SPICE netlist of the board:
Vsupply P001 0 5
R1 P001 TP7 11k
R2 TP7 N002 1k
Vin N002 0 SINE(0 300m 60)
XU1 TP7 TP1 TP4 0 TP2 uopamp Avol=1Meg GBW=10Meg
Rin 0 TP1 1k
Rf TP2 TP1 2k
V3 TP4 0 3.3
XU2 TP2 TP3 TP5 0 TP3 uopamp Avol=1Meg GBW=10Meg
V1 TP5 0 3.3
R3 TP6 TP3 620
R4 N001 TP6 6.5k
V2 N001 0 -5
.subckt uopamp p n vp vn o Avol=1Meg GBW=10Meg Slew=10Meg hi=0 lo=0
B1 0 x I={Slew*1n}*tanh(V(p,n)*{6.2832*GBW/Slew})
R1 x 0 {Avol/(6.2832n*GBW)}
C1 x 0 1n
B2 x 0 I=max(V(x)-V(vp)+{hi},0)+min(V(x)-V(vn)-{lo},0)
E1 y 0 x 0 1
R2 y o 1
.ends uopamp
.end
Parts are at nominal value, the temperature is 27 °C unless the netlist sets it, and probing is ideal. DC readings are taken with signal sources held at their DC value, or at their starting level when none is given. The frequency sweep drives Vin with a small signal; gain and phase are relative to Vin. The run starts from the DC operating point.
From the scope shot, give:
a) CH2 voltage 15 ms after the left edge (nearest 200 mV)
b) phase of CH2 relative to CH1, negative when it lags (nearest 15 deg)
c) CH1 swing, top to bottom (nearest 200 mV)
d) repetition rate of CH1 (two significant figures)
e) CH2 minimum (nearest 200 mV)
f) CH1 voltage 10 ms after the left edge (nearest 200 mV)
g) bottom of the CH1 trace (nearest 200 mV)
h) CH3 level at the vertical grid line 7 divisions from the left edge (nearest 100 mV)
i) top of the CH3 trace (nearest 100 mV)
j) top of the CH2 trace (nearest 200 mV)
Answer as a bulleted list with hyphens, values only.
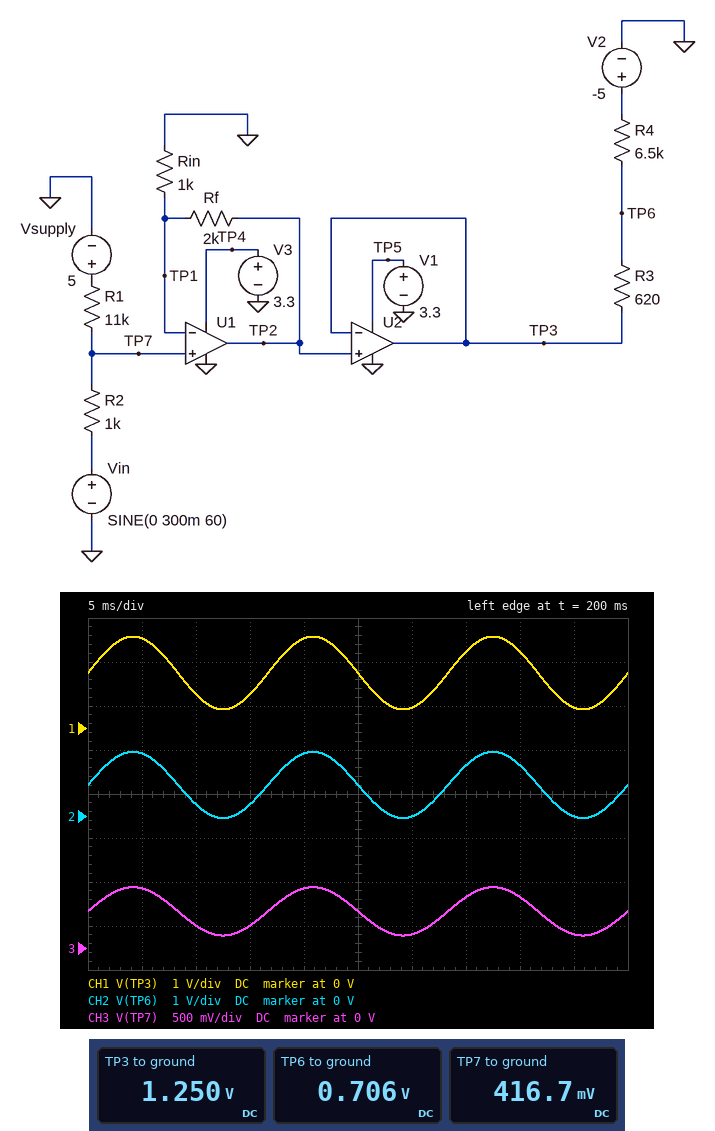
- 200 mV
- 0 deg
- 1.6 V
- 60 Hz
- 0 V
- 800 mV
- 400 mV
- 600 mV
- 700 mV
- 1.4 V
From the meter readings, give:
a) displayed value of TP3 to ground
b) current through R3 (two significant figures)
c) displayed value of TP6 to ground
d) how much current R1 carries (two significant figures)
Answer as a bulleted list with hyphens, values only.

- 1.250 V
- 880 µA
- 0.706 V
- 420 µA
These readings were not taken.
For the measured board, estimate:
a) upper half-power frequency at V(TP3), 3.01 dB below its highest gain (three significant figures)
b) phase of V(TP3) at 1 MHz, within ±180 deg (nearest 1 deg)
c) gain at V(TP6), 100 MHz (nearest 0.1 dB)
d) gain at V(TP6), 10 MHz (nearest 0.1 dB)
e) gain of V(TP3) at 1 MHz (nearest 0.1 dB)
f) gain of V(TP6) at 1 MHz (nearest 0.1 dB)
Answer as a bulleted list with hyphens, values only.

- 3.04 MHz
- -22 deg
- -41.6 dB
- -5.0 dB
- 8.4 dB
- 7.6 dB
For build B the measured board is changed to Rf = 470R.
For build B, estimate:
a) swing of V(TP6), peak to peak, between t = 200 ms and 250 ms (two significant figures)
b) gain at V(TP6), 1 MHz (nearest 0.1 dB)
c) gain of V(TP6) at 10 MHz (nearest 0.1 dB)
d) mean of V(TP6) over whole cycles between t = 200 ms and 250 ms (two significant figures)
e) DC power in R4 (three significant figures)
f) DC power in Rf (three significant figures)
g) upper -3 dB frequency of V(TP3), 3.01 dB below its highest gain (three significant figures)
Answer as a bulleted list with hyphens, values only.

- 740 mV
- 1.7 dB
- -6.2 dB
- 120 mV
- 4.04 mW
- 81.6 µW
- 5.17 MHz
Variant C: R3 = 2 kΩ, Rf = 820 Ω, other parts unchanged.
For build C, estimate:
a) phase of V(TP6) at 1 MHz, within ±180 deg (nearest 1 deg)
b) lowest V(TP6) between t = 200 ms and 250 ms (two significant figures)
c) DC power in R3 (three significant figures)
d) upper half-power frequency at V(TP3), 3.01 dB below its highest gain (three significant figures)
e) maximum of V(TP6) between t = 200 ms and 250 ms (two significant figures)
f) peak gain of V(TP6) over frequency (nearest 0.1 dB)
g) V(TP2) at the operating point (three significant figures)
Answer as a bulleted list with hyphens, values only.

- -16 deg
- -980 mV
- 918 µW
- 4.48 MHz
- -210 mV
- 2.1 dB
- 758 mV
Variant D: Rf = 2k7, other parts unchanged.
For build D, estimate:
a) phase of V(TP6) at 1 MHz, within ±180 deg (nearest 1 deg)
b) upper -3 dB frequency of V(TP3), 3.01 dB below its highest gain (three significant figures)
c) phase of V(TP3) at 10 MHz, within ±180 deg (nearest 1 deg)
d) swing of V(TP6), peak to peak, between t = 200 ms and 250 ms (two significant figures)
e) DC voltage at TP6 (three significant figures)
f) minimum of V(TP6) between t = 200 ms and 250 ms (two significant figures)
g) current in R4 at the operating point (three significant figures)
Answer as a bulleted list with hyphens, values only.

- -26 deg
- 2.53 MHz
- -120 deg
- 1.9 V
- 972 mV
- 43 mV
- 919 µA
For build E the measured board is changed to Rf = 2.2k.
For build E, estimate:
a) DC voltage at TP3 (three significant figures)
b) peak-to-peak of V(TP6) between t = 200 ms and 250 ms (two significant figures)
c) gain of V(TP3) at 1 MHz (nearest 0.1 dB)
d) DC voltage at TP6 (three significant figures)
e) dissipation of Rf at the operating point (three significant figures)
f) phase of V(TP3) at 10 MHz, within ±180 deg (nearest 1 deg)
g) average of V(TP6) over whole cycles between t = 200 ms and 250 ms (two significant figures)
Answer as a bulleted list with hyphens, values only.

- 1.33 V
- 1.6 V
- 8.9 dB
- 782 mV
- 382 µW
- -118 deg
- 780 mV
